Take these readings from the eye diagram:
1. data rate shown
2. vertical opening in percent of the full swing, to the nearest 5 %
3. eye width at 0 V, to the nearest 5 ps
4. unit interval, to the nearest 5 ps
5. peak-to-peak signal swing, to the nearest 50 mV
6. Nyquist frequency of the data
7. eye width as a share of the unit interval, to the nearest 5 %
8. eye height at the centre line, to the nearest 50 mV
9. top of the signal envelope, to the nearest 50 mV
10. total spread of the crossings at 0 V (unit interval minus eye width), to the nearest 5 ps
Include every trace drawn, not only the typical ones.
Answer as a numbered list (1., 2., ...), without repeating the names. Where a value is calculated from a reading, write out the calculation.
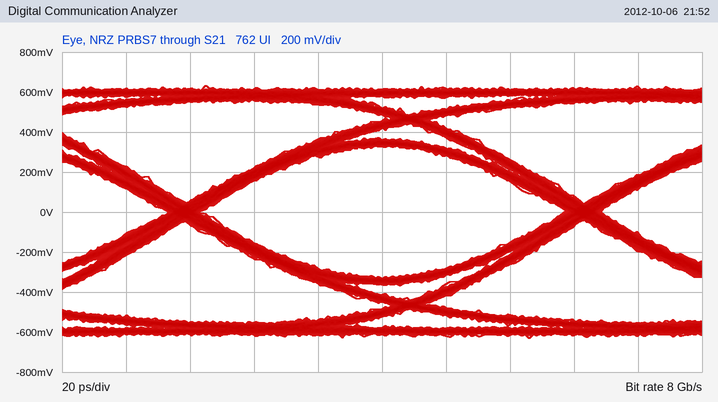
1. 8 Gb/s
2. 650 mV / 1.25 V ≈ 52.0 %, so 50 % to the nearest 5 %
3. 115 ps
4. 125 ps
5. 1.25 V
6. 4 GHz
7. 115 ps / 125 ps ≈ 92.0 %, so 90 % to the nearest 5 %
8. 650 mV
9. 650 mV
10. 10 ps
